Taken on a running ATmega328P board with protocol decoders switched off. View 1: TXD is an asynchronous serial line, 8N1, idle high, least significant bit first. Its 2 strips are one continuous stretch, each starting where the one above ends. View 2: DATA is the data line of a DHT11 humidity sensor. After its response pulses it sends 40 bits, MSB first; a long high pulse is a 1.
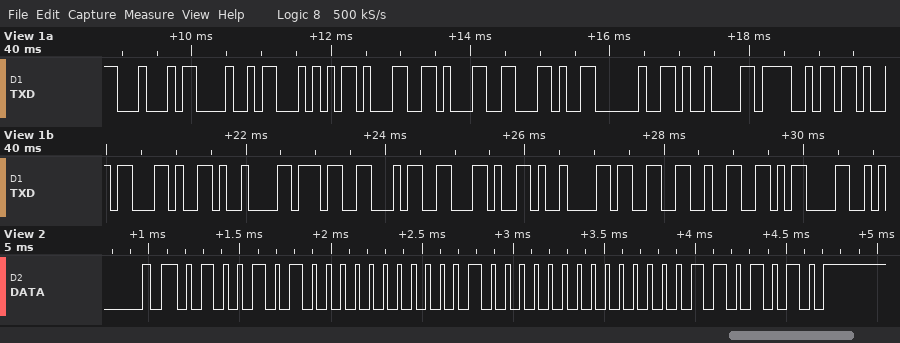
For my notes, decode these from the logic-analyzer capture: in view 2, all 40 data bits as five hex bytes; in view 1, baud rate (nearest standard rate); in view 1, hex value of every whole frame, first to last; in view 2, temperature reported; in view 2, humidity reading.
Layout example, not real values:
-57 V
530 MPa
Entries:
4A 00 20 00 6A
9600 baud
44 48 54 31 31 2C 20 09 4F 4B 2C 09 37 34 2C 09 33 32 0D
32.0 °C
74 %
